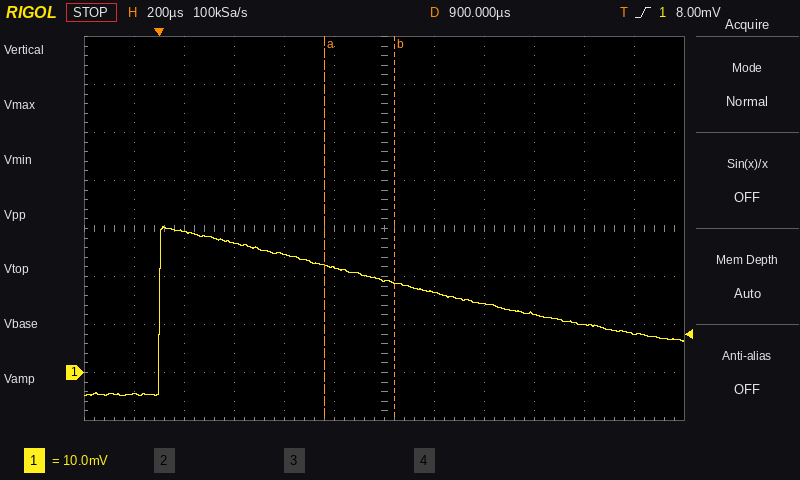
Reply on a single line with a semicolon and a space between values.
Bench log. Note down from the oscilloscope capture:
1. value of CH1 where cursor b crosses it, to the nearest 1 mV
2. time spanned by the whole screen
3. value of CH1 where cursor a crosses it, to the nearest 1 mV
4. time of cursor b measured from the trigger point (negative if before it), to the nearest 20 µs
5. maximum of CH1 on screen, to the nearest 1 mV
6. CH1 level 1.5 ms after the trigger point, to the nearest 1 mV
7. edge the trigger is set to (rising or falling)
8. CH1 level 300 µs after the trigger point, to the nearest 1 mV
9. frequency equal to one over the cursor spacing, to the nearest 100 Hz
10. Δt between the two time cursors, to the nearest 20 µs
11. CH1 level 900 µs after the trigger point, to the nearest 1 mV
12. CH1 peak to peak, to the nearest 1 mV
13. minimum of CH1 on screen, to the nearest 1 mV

19 mV; 2.4 ms; 22 mV; +940 µs; 30 mV; 12 mV; rising; 27 mV; 3.6 kHz; 280 µs; 19 mV; 35 mV; -5 mV
